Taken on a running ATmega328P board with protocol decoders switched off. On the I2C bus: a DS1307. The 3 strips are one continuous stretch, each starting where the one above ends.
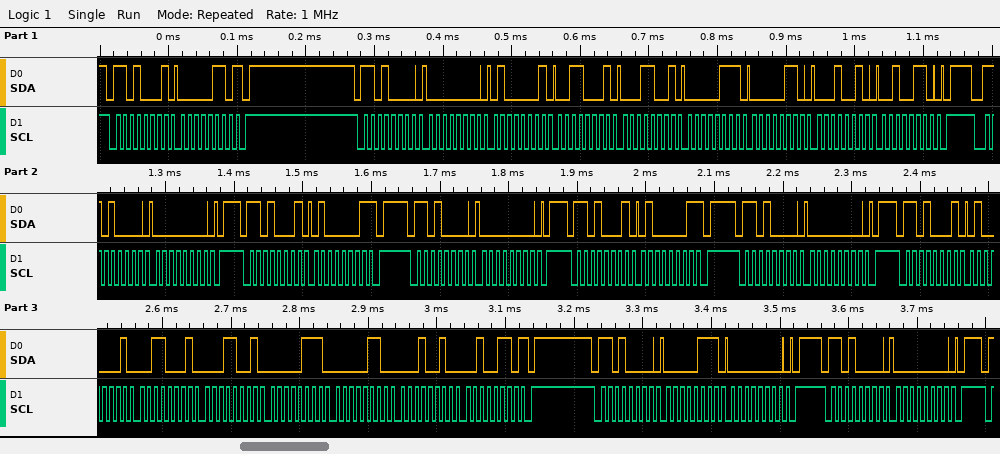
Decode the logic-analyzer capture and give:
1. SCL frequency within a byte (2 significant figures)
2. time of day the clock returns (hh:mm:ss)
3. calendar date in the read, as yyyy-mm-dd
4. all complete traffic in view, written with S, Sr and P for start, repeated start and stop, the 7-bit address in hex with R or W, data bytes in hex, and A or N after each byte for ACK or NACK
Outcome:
100 kHz
19:31:41
2026-12-06
S 68R A 06 N P S 68W A 00 A 41 A 31 A 19 A 07 A 06 A 12 A 26 A P S 68W A 00 A P S 68R A 41 N P S 68W A 00 A P S 68R A 41 N P S 68W A 00 A P S 68R A 41 A 31 A 19 A 07 A 06 A 12 A 26 N P S 68W A 07 A 00 A P S 68W A 00 A P
